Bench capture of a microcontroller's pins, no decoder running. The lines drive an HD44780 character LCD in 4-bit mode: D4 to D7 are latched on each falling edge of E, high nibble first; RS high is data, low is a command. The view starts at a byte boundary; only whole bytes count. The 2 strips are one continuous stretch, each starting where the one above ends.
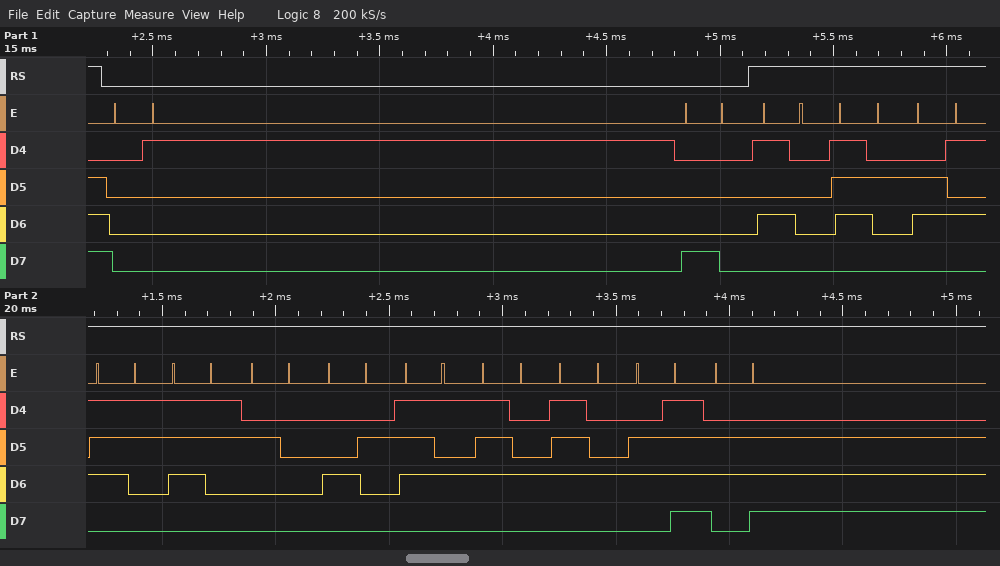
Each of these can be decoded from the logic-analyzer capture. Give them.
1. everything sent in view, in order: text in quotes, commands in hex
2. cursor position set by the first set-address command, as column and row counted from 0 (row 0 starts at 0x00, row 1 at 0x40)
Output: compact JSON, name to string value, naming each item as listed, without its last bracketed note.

{"everything sent in view, in order: text in quotes, commands in hex": "0x01 0x80 \"Press Button\"", "cursor position set by the first set-address command, as column and row counted from 0": "column 0, row 0"}
